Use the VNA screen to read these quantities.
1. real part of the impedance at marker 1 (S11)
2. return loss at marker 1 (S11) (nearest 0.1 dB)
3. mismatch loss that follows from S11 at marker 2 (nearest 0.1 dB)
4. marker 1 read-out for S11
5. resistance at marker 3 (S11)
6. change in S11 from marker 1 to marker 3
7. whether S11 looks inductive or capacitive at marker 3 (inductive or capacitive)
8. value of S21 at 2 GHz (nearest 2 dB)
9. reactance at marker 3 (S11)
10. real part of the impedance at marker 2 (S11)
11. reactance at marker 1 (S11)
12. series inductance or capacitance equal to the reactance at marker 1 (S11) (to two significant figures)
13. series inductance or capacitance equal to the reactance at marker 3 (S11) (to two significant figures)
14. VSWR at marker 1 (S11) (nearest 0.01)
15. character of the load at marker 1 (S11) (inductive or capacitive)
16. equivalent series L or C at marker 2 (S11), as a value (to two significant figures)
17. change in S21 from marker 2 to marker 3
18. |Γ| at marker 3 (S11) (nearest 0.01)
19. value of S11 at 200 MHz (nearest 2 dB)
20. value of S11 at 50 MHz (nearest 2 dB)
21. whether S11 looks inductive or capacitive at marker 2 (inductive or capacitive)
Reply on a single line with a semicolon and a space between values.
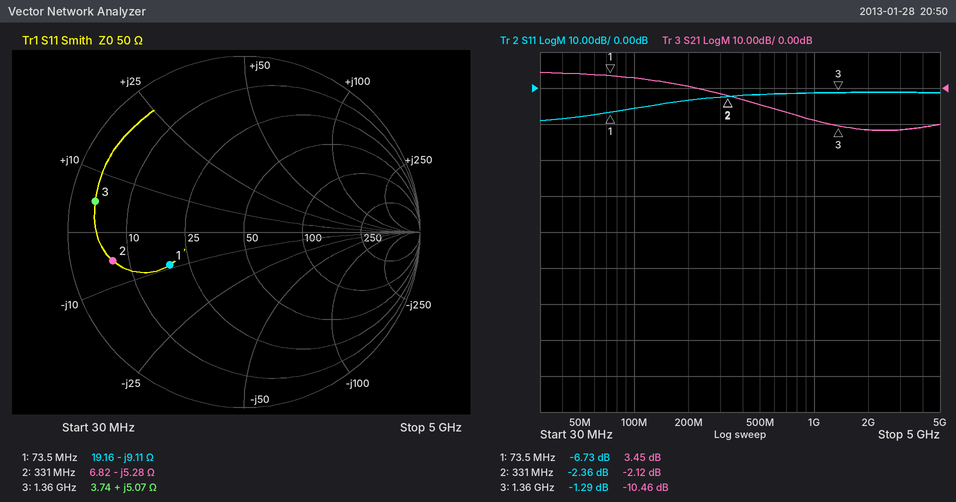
19.16 Ω; 6.7 dB; 3.8 dB; -6.73 dB; 3.74 Ω; 5.44 dB; inductive; -12 dB; +5.07 Ω; 6.82 Ω; -9.11 Ω; 240 pF; 590 pH; 2.71; capacitive; 91 pF; -8.34 dB; 0.86; -4 dB; -8 dB; capacitive
